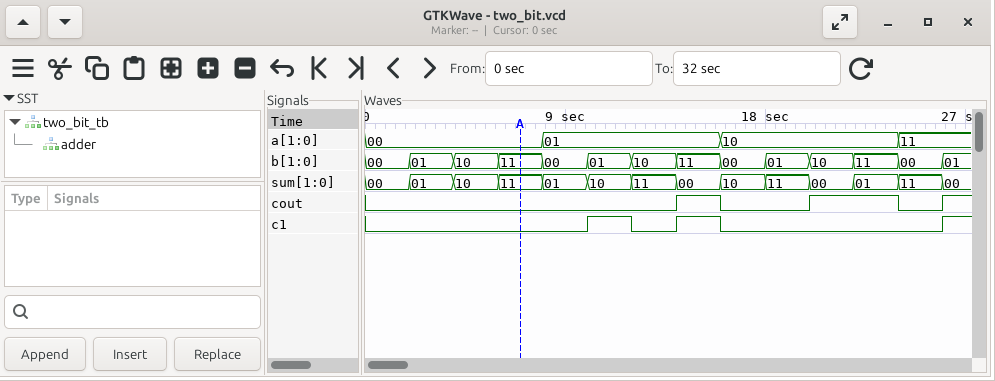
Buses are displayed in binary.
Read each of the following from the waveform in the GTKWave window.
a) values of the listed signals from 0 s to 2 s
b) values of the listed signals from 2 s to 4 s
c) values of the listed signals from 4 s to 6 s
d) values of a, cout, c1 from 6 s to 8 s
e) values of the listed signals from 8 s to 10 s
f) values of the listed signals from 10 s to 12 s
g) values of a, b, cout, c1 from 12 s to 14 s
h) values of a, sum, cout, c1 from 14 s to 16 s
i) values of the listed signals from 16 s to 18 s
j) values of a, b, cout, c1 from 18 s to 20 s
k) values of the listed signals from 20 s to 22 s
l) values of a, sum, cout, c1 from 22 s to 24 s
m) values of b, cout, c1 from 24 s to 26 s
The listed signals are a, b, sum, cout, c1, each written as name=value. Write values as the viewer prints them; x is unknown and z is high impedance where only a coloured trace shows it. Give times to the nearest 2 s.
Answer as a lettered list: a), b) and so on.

a) a=00, b=00, sum=00, cout=0, c1=0
b) a=00, b=01, sum=01, cout=0, c1=0
c) a=00, b=10, sum=10, cout=0, c1=0
d) a=00, cout=0, c1=0
e) a=01, b=00, sum=01, cout=0, c1=0
f) a=01, b=01, sum=10, cout=0, c1=1
g) a=01, b=10, cout=0, c1=0
h) a=01, sum=00, cout=1, c1=1
i) a=10, b=00, sum=10, cout=0, c1=0
j) a=10, b=01, cout=0, c1=0
k) a=10, b=10, sum=00, cout=1, c1=0
l) a=10, sum=01, cout=1, c1=0
m) b=00, cout=0, c1=0
